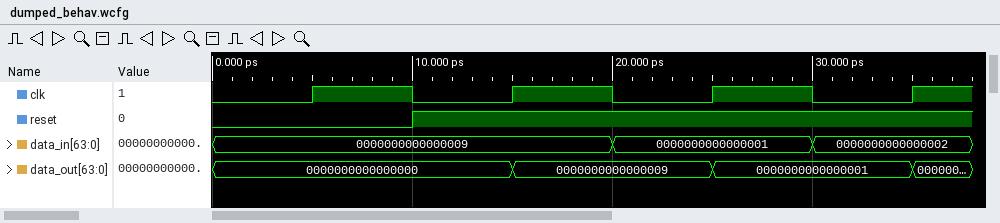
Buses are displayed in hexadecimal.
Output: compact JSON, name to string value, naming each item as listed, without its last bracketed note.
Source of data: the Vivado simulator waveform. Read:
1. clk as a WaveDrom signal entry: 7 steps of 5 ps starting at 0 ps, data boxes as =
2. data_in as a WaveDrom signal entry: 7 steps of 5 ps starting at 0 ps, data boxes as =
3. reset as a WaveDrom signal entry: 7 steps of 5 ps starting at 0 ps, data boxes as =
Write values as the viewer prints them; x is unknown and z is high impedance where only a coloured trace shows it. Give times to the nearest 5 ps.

{"clk as a WaveDrom signal entry: 7 steps of 5 ps starting at 0 ps, data boxes as =": "{name: 'clk', wave: '0101010'}", "data_in as a WaveDrom signal entry: 7 steps of 5 ps starting at 0 ps, data boxes as =": "{name: 'data_in', wave: '=...=.=', data: '0000000000000009 0000000000000001 0000000000000002'}", "reset as a WaveDrom signal entry: 7 steps of 5 ps starting at 0 ps, data boxes as =": "{name: 'reset', wave: '0.1....'}"}
